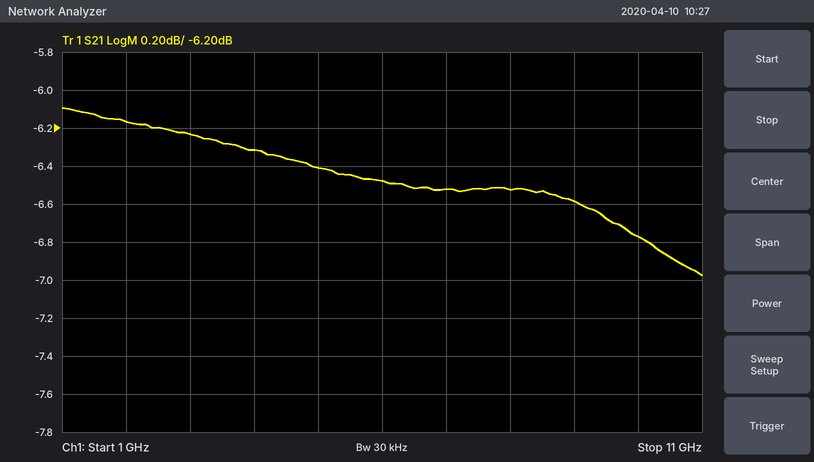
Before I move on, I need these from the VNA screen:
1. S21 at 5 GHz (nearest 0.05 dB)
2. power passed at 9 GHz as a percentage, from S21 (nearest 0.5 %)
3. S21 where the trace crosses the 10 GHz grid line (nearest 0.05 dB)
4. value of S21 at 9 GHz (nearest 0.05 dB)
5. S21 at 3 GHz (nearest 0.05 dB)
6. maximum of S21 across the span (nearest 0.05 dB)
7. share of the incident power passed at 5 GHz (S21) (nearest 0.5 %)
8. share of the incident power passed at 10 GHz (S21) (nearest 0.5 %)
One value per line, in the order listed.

-6.40 dB
22.0 %
-6.75 dB
-6.60 dB
-6.25 dB
-6.10 dB
23.0 %
21.0 %
